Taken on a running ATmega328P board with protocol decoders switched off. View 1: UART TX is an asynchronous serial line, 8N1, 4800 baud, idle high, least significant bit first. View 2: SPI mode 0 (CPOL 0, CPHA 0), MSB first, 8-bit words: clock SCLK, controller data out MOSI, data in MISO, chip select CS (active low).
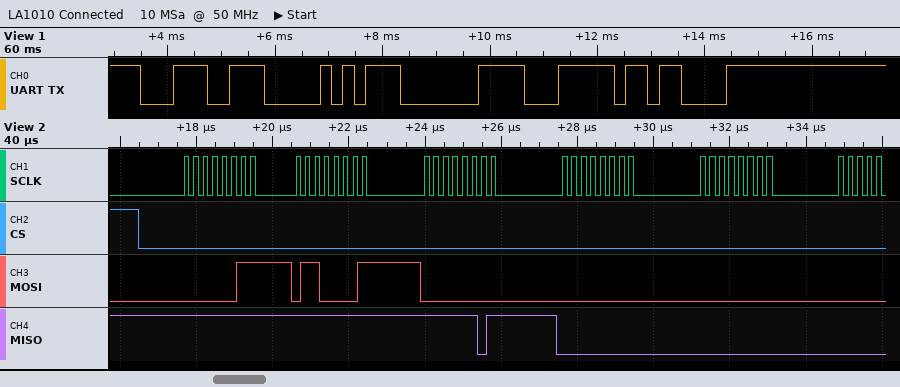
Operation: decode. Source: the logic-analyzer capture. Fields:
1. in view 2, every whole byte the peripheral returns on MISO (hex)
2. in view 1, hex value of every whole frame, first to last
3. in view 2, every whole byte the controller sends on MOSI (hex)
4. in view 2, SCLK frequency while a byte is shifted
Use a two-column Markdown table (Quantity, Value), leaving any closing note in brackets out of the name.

| Quantity | Value |
|---|---|
| in view 2, every whole byte the peripheral returns on MISO | 0xFF 0xFF 0xFD 0x00 0x00 |
| in view 1, hex value of every whole frame, first to last | 9C 50 C0 7C C3 |
| in view 2, every whole byte the controller sends on MOSI | 0x03 0x61 0x00 0x00 0x00 |
| in view 2, SCLK frequency while a byte is shifted | 4 MHz |
